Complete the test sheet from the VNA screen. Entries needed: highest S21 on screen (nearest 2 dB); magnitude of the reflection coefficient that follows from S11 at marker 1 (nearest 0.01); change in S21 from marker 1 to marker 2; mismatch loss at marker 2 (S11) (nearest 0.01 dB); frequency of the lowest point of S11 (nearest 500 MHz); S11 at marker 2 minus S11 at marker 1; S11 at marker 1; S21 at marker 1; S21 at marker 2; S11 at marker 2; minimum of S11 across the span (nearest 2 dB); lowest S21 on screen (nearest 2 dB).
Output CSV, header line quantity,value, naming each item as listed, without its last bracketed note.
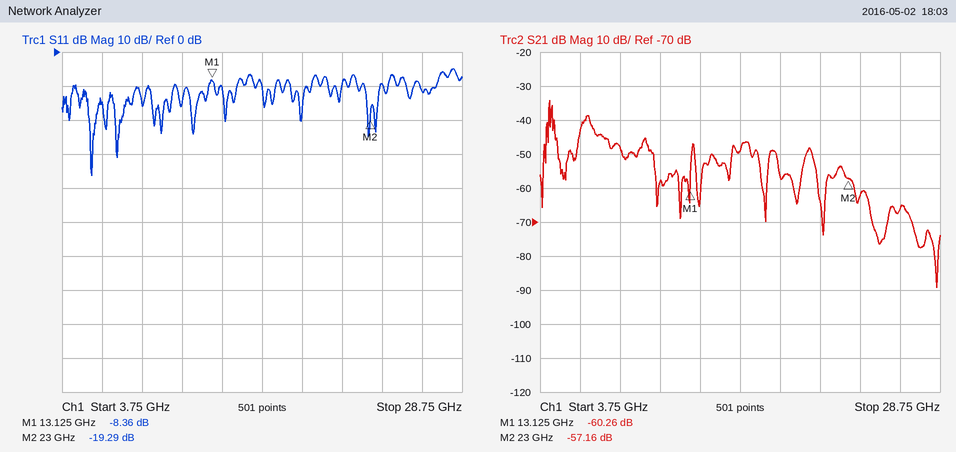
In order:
quantity,value
highest S21 on screen,-34 dB
magnitude of the reflection coefficient that follows from S11 at marker 1,0.38
change in S21 from marker 1 to marker 2,3.10 dB
mismatch loss at marker 2 (S11),0.05 dB
frequency of the lowest point of S11,5.5 GHz
S11 at marker 2 minus S11 at marker 1,-10.93 dB
S11 at marker 1,-8.36 dB
S21 at marker 1,-60.26 dB
S21 at marker 2,-57.16 dB
S11 at marker 2,-19.29 dB
minimum of S11 across the span,-36 dB
lowest S21 on screen,-90 dB
